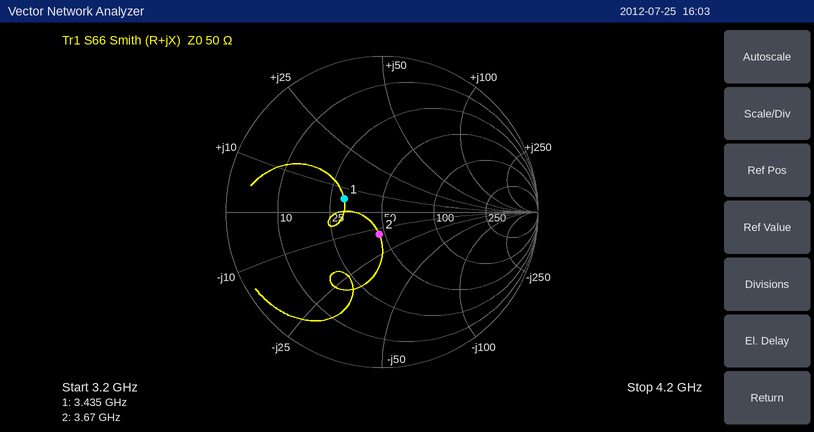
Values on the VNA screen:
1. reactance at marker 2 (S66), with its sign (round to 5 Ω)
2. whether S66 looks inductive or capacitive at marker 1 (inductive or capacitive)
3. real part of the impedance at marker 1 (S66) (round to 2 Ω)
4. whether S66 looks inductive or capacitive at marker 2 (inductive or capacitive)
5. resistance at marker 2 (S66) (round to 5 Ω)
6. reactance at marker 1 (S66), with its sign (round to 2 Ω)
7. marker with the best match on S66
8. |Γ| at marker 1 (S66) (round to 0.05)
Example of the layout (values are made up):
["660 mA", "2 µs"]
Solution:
["-15 Ω", "inductive", "30 Ω", "capacitive", "45 Ω", "+6 Ω", "marker 2", "0.25"]
